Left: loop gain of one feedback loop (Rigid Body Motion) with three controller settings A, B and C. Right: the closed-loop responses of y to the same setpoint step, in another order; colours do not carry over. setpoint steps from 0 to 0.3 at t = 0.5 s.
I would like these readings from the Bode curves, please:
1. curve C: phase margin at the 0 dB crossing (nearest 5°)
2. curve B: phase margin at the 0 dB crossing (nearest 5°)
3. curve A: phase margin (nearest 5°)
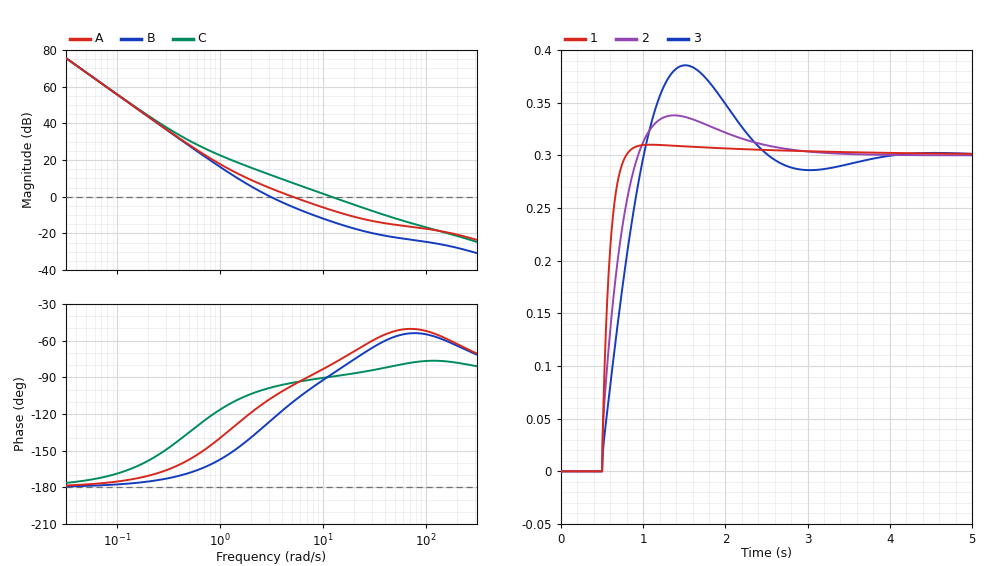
90°
55°
85°
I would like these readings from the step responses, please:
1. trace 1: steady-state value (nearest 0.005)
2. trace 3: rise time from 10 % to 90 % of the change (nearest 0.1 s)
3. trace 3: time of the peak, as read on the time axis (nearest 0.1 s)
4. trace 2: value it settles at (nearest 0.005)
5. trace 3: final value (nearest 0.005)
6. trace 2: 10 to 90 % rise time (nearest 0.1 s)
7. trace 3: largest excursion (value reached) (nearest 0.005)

0.300
0.4 s
1.5 s
0.300
0.300
0.3 s
0.385
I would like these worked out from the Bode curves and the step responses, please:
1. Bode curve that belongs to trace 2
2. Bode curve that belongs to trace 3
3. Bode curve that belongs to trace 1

A
B
C
